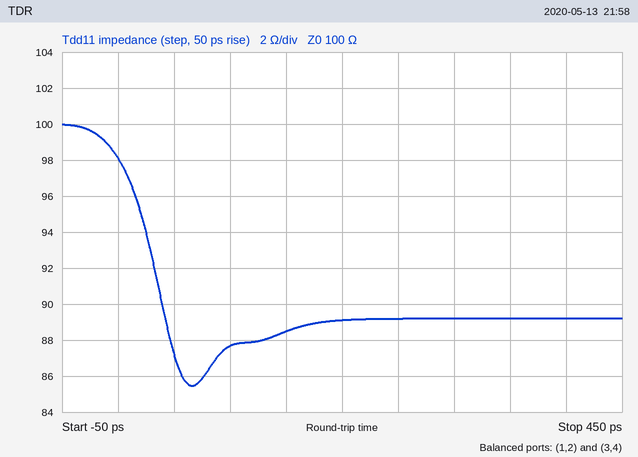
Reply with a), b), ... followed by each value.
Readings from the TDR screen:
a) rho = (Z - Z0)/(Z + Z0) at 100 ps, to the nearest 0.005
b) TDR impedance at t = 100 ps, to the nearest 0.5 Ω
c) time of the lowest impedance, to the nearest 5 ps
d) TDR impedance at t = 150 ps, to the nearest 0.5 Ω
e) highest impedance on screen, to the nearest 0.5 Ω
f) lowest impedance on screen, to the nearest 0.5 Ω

a) -0.065
b) 87.5 Ω
c) 65 ps
d) 88.5 Ω
e) 100.0 Ω
f) 85.5 Ω
